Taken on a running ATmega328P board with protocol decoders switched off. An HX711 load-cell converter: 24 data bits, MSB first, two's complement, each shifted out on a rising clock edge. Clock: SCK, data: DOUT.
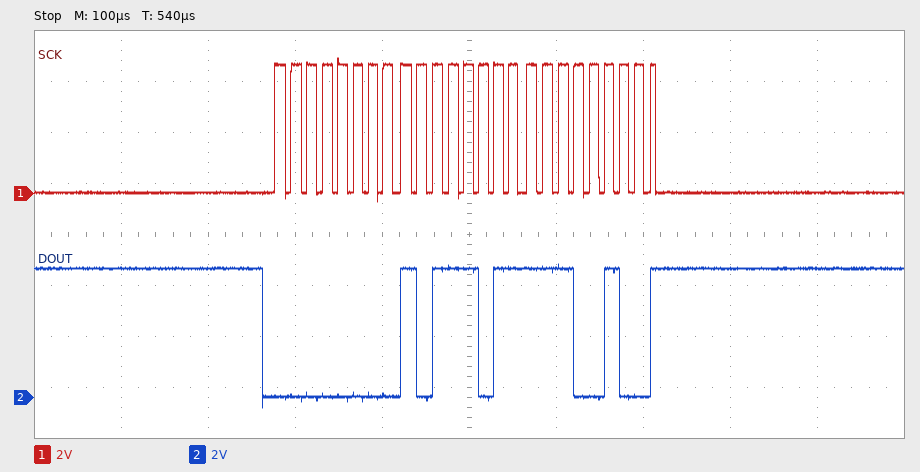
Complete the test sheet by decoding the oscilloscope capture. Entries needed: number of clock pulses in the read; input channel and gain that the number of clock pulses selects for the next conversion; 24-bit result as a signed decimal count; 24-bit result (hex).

25
channel A, gain 128
48100
0x00BBE4
